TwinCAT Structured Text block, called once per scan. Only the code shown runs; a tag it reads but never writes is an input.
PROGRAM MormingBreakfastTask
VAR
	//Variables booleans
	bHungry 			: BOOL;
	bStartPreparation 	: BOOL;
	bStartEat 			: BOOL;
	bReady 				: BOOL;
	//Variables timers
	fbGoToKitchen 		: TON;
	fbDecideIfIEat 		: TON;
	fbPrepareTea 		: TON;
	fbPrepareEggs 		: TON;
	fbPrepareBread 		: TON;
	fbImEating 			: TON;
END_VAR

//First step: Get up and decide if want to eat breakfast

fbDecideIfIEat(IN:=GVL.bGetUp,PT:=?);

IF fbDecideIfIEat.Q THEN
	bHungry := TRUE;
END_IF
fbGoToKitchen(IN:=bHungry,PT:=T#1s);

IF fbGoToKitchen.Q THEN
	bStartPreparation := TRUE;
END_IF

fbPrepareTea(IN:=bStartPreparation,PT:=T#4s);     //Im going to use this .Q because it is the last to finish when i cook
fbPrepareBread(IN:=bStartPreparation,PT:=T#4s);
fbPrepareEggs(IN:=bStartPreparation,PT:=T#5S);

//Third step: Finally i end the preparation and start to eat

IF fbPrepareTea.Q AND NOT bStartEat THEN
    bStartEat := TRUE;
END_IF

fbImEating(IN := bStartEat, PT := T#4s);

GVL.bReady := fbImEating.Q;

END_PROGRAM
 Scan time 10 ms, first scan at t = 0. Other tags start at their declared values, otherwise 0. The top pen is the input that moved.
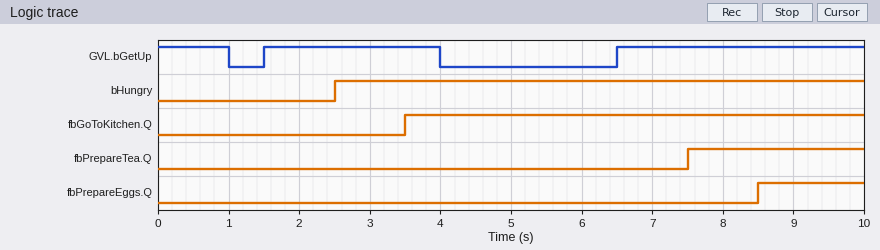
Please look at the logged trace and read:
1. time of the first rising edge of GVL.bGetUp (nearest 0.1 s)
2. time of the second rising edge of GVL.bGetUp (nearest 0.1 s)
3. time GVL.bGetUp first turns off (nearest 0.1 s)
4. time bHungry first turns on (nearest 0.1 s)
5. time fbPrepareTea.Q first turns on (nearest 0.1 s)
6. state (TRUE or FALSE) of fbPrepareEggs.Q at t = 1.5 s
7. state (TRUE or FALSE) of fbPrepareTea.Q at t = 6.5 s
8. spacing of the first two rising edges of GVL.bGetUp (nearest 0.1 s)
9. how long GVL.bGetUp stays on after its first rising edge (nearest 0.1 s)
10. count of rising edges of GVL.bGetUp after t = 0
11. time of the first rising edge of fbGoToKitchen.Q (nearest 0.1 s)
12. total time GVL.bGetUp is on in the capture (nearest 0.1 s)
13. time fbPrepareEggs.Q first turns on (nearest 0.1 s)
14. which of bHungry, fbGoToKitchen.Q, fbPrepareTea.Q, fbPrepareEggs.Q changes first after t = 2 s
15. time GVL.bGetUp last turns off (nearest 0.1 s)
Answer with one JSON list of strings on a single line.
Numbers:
["1.5 s", "6.5 s", "1.0 s", "2.5 s", "7.5 s", "FALSE", "FALSE", "5.0 s", "2.5 s", "2", "3.5 s", "7.0 s", "8.5 s", "bHungry", "4.0 s"]
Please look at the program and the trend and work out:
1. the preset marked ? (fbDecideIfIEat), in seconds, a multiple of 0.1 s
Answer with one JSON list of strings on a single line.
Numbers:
["1.0 s"]
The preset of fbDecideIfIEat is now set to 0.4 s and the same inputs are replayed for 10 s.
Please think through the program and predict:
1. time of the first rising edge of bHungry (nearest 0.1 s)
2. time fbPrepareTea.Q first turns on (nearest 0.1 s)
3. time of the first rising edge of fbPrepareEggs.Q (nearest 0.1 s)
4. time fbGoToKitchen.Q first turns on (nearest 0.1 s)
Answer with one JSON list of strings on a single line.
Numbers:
["0.4 s", "5.4 s", "6.4 s", "1.4 s"]
